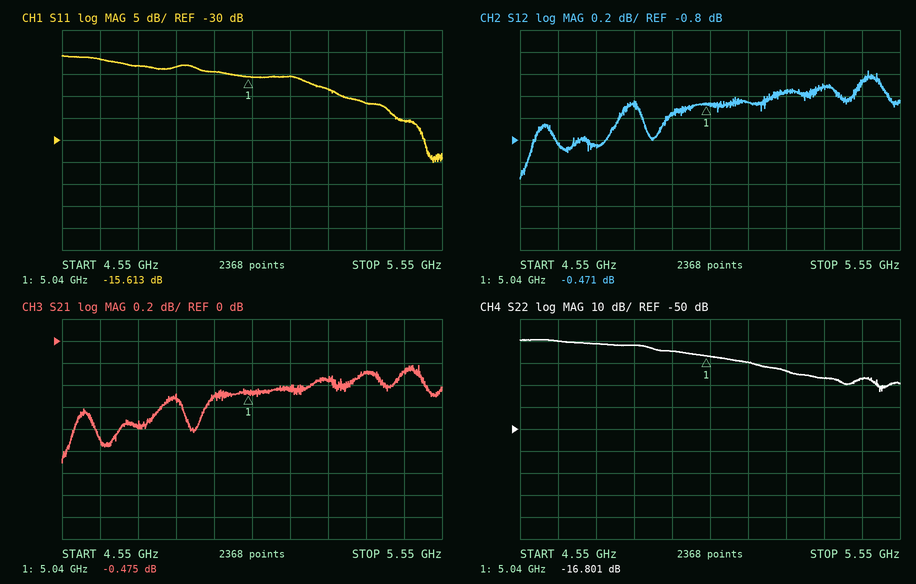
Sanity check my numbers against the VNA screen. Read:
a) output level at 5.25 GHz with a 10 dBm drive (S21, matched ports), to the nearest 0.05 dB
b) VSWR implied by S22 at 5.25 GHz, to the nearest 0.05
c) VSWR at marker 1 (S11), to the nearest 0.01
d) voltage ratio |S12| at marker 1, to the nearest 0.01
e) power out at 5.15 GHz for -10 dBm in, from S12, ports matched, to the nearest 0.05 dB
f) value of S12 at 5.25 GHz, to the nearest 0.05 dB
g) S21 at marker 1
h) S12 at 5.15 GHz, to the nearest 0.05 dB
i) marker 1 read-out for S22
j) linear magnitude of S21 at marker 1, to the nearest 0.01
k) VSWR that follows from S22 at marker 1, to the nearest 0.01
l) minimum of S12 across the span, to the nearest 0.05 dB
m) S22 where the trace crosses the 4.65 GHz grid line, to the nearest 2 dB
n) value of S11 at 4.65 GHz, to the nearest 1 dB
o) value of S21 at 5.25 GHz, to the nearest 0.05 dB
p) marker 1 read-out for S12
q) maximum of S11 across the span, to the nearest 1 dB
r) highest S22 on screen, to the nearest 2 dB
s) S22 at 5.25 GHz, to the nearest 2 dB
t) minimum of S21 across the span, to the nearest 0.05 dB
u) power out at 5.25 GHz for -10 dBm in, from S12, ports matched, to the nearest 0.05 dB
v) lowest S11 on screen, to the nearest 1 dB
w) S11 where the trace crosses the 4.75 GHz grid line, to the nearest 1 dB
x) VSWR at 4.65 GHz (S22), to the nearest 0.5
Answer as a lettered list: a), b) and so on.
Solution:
a) 9.65 dBm
b) 1.15
c) 1.40
d) 0.95
e) -10.45 dBm
f) -0.35 dB
g) -0.475 dB
h) -0.45 dB
i) -16.801 dB
j) 0.95
k) 1.34
l) -1.15 dB
m) -10 dB
n) -12 dB
o) -0.35 dB
p) -0.471 dB
q) -11 dB
r) -10 dB
s) -24 dB
t) -1.10 dB
u) -10.35 dBm
v) -35 dB
w) -13 dB
x) 2.0
